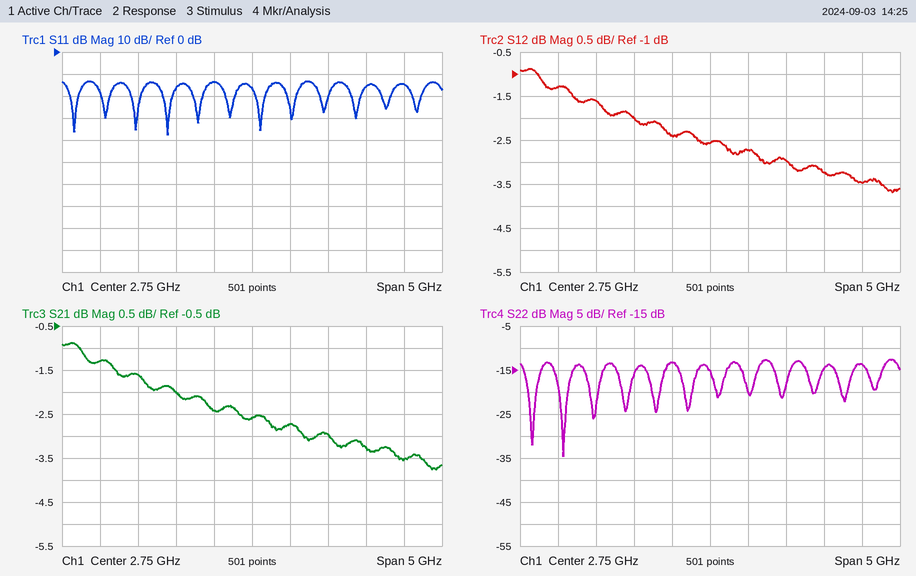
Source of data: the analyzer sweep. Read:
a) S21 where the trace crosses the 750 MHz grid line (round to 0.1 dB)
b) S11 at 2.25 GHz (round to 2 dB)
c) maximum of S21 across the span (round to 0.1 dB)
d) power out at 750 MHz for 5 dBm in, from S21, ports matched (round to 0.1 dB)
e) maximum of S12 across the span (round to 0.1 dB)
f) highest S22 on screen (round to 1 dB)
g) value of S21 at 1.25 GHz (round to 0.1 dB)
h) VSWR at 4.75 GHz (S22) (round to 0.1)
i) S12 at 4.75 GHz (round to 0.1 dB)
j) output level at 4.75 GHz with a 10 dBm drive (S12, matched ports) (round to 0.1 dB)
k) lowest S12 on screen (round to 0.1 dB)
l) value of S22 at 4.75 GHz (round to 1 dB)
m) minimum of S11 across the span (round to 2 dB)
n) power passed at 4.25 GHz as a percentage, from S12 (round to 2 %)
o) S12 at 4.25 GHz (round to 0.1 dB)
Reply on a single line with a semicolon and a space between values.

-1.3 dB; -14 dB; -0.9 dB; 3.7 dBm; -0.9 dB; -13 dB; -1.6 dB; 1.5; -3.5 dB; 6.5 dBm; -3.7 dB; -14 dB; -38 dB; 48 %; -3.2 dB
